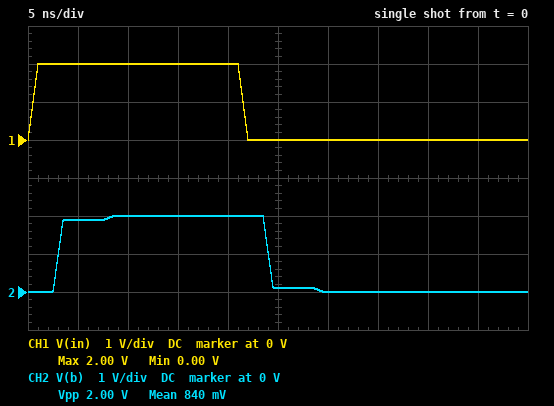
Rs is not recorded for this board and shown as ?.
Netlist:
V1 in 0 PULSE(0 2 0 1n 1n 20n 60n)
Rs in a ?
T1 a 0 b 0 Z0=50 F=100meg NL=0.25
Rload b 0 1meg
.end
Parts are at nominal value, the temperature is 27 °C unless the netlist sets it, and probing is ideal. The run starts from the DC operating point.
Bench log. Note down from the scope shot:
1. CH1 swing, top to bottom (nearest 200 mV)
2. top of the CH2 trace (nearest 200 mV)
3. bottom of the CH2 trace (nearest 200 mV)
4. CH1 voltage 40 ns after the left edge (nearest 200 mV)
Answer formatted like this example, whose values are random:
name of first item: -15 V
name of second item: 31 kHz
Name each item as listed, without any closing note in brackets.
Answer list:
CH1 swing, top to bottom: 2.0 V
top of the CH2 trace: 2.0 V
bottom of the CH2 trace: 0 V
CH1 voltage 40 ns after the left edge: 0 V
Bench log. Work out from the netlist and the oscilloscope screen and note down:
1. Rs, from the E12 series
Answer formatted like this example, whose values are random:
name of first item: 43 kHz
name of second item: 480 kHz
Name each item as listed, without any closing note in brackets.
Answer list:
Rs, from the E12 series: 56 Ω
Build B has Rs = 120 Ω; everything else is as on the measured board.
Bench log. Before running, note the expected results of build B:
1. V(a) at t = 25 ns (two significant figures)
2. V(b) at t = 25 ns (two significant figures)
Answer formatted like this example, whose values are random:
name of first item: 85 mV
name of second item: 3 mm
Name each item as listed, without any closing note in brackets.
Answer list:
V(a) at t = 25 ns: 1.4 V
V(b) at t = 25 ns: 800 mV
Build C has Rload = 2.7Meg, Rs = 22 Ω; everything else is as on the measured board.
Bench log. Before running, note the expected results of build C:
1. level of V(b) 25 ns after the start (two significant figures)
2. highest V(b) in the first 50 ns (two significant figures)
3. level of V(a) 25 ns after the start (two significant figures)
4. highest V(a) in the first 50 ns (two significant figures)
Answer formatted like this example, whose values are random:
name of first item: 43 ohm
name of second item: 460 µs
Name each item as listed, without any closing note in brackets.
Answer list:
level of V(b) 25 ns after the start: -760 mV
highest V(b) in the first 50 ns: 2.8 V
level of V(a) 25 ns after the start: 600 mV
highest V(a) in the first 50 ns: 2.2 V
